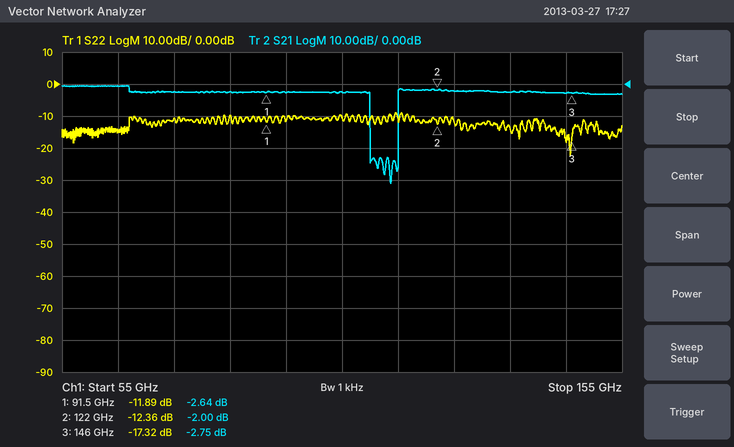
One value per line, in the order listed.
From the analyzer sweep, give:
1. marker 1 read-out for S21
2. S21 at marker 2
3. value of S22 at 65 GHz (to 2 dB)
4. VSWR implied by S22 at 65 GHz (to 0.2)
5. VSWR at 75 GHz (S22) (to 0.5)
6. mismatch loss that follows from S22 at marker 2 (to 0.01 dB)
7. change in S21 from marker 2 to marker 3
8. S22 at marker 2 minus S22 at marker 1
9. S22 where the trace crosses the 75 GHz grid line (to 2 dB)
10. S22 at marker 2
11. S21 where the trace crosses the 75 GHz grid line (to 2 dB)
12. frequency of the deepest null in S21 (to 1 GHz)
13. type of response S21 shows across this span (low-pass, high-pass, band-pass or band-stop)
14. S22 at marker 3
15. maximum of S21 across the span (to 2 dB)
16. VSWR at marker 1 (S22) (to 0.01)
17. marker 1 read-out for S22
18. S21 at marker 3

-2.64 dB
-2.00 dB
-14 dB
1.4
2.0
0.26 dB
-0.75 dB
-0.47 dB
-10 dB
-12.36 dB
-2 dB
114 GHz
band-stop
-17.32 dB
0 dB
1.68
-11.89 dB
-2.75 dB
